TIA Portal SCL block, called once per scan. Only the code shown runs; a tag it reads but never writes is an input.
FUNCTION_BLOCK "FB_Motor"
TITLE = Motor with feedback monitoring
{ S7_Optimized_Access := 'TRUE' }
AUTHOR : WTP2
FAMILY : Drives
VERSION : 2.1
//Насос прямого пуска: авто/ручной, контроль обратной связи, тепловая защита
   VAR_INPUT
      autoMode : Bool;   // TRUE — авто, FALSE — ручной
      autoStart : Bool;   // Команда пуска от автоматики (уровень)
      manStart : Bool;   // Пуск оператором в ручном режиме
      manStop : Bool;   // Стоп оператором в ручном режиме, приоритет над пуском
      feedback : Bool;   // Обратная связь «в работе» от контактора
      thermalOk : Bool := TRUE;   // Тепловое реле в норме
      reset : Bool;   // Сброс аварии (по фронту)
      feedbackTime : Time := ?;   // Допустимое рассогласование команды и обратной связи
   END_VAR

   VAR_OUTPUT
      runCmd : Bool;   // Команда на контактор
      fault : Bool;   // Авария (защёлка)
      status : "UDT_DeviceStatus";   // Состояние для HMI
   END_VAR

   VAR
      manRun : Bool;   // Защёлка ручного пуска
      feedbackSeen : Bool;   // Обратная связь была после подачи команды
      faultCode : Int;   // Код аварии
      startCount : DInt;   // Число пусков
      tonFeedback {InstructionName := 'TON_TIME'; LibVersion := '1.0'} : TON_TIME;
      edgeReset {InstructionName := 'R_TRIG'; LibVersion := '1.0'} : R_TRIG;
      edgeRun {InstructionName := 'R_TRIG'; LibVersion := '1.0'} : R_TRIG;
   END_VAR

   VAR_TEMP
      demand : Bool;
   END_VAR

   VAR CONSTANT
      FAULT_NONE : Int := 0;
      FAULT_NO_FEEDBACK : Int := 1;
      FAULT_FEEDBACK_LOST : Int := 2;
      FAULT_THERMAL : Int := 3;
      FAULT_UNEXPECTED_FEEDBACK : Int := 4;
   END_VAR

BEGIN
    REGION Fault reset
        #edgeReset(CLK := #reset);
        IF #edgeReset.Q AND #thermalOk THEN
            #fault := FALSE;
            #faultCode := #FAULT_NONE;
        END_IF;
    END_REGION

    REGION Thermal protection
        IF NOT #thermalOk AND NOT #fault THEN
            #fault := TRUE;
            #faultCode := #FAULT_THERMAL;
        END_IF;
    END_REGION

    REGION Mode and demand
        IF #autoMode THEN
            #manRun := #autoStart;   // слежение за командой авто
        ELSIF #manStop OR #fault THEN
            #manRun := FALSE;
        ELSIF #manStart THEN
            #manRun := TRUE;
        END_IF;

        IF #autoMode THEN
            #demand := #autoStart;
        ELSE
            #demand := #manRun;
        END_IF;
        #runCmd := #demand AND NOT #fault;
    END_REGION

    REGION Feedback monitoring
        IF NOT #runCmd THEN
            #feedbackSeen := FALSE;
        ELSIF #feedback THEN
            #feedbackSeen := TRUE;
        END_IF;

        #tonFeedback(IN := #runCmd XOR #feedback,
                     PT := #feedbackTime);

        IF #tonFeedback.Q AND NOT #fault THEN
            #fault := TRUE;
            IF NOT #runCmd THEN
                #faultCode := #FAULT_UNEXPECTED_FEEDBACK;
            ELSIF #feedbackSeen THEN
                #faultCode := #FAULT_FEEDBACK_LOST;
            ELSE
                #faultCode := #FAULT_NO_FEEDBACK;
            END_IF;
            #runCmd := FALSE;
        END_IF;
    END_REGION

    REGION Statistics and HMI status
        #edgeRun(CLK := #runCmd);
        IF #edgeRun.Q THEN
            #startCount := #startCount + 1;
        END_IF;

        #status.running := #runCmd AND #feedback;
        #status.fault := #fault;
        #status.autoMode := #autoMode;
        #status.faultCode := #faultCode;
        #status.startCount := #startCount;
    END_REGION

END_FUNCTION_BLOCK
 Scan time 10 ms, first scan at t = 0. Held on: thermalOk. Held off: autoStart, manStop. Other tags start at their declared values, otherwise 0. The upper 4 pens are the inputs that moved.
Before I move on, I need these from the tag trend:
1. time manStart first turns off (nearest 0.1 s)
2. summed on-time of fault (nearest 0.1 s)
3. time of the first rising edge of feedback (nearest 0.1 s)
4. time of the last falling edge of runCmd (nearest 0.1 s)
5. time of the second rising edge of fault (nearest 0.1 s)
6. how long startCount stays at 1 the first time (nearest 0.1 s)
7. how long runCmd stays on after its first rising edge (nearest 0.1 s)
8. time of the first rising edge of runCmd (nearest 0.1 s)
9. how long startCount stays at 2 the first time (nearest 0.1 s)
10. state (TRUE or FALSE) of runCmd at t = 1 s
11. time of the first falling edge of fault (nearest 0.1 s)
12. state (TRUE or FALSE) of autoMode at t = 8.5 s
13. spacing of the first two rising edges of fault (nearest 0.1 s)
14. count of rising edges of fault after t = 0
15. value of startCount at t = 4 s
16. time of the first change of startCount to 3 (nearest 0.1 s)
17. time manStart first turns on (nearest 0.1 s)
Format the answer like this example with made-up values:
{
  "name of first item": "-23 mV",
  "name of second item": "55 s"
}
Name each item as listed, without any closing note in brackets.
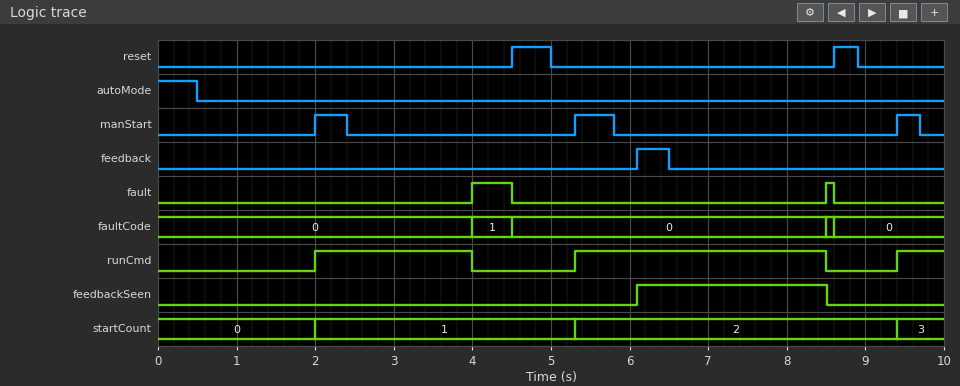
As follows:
{
  "time manStart first turns off": "2.4 s",
  "summed on-time of fault": "0.6 s",
  "time of the first rising edge of feedback": "6.1 s",
  "time of the last falling edge of runCmd": "8.5 s",
  "time of the second rising edge of fault": "8.5 s",
  "how long startCount stays at 1 the first time": "3.3 s",
  "how long runCmd stays on after its first rising edge": "2.0 s",
  "time of the first rising edge of runCmd": "2.0 s",
  "how long startCount stays at 2 the first time": "4.1 s",
  "state (TRUE or FALSE) of runCmd at t = 1 s": "FALSE",
  "time of the first falling edge of fault": "4.5 s",
  "state (TRUE or FALSE) of autoMode at t = 8.5 s": "FALSE",
  "spacing of the first two rising edges of fault": "4.5 s",
  "count of rising edges of fault after t = 0": "2",
  "value of startCount at t = 4 s": "1",
  "time of the first change of startCount to 3": "9.4 s",
  "time manStart first turns on": "2.0 s"
}
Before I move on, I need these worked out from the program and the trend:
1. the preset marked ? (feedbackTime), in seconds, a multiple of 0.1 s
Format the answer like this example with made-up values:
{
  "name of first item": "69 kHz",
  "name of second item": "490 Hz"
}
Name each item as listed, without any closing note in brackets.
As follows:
{
  "the preset marked ? (feedbackTime), in seconds, a multiple of 0.1 s": "2.0 s"
}
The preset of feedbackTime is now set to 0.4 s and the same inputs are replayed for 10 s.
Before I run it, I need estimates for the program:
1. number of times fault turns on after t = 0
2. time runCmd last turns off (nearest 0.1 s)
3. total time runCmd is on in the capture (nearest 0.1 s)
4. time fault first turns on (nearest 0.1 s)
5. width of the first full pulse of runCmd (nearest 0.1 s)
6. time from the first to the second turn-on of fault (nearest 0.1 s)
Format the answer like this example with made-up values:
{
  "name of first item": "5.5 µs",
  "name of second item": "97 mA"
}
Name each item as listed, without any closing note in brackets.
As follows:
{
  "number of times fault turns on after t = 0": "3",
  "time runCmd last turns off": "9.8 s",
  "total time runCmd is on in the capture": "1.2 s",
  "time fault first turns on": "2.4 s",
  "width of the first full pulse of runCmd": "0.4 s",
  "time from the first to the second turn-on of fault": "3.3 s"
}
